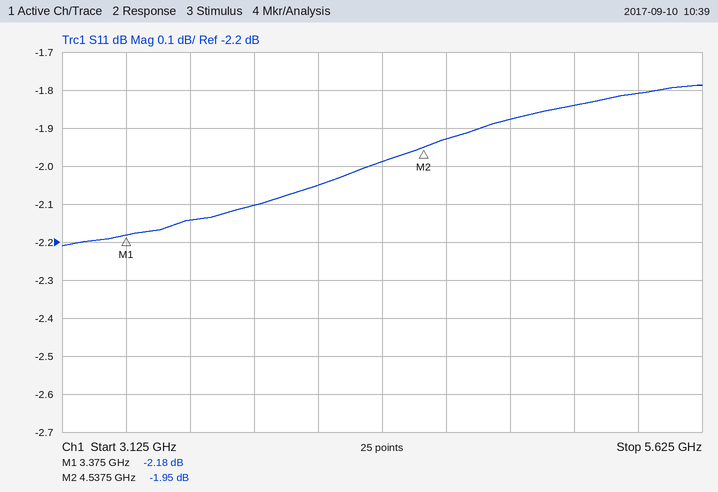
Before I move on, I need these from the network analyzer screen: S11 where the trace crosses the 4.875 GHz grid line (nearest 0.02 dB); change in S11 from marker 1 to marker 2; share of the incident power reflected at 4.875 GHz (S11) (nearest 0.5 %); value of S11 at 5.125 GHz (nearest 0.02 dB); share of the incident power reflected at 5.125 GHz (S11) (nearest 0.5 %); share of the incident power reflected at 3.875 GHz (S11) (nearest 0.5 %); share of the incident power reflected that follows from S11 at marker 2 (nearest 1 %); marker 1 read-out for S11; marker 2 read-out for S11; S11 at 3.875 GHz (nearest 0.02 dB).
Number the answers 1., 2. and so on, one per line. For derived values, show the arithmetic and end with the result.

1. -1.88 dB
2. -1.95 − (-2.18) = 0.23 dB
3. 10^(-1.88/10) ≈ 64.9 %, so 65.0 % to the nearest 0.5 %
4. -1.84 dB
5. 10^(-1.84/10) ≈ 65.5 %
6. 10^(-2.1/10) ≈ 61.7 %, so 61.5 % to the nearest 0.5 %
7. 10^(-1.95/10) ≈ 64 %
8. -2.18 dB
9. -1.95 dB
10. -2.10 dB
